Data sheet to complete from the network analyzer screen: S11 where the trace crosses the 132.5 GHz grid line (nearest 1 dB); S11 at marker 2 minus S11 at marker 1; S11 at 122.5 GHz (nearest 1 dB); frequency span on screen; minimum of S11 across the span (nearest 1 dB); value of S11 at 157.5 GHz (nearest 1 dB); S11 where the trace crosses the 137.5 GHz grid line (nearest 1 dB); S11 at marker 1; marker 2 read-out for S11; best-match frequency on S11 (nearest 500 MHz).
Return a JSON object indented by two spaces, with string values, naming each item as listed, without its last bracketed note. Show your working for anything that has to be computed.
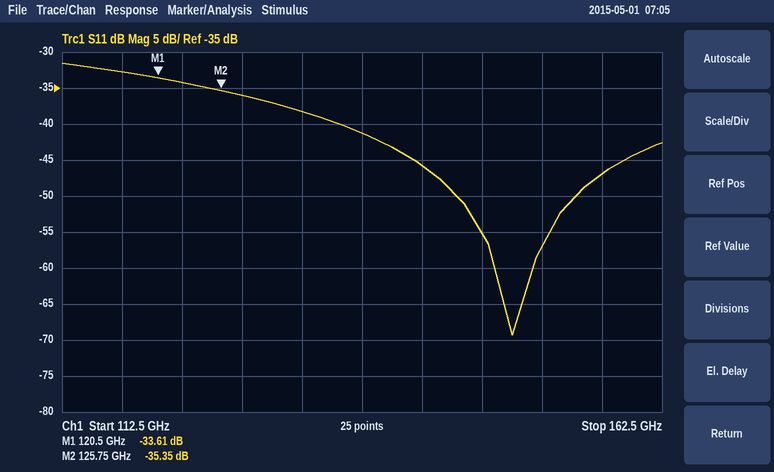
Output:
{
  "S11 where the trace crosses the 132.5 GHz grid line": "-38 dB",
  "S11 at marker 2 minus S11 at marker 1": "-35.35 − (-33.61) = -1.74 dB",
  "S11 at 122.5 GHz": "-34 dB",
  "frequency span on screen": "50 GHz",
  "minimum of S11 across the span": "-69 dB",
  "value of S11 at 157.5 GHz": "-47 dB",
  "S11 where the trace crosses the 137.5 GHz grid line": "-41 dB",
  "S11 at marker 1": "-33.61 dB",
  "marker 2 read-out for S11": "-35.35 dB",
  "best-match frequency on S11": "150.0 GHz"
}
